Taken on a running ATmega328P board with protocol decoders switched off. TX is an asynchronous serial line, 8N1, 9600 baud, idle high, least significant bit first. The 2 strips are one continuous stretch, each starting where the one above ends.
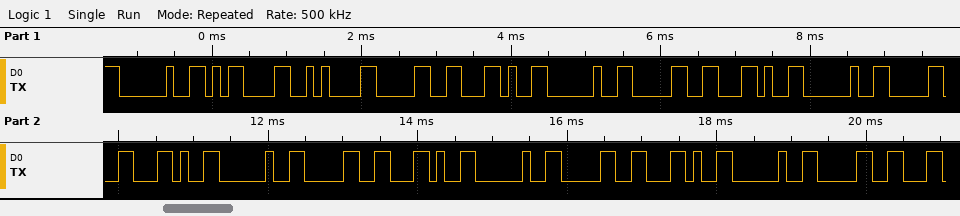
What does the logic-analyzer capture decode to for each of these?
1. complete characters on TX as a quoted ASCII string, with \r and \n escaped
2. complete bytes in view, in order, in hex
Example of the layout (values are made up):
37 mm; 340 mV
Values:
" \r\n0, 0, 0, 0, 0, 0"; 20 0D 0A 30 2C 20 30 2C 20 30 2C 20 30 2C 20 30 2C 20 30
